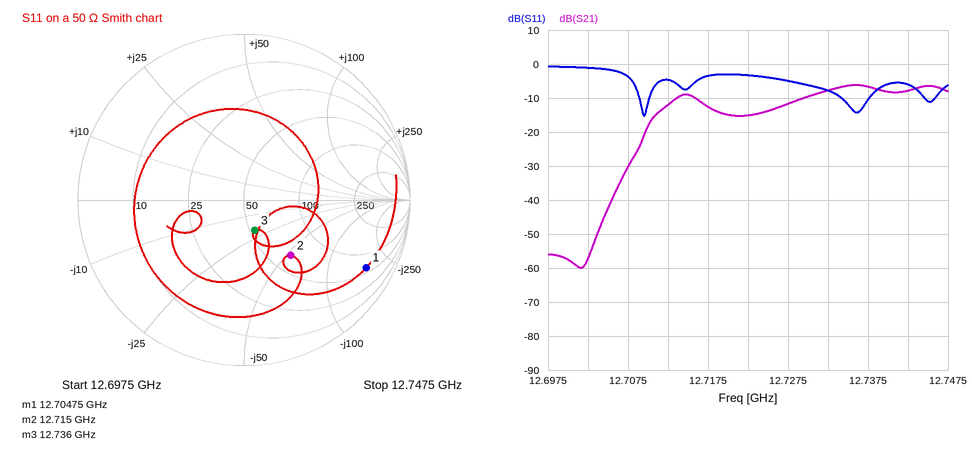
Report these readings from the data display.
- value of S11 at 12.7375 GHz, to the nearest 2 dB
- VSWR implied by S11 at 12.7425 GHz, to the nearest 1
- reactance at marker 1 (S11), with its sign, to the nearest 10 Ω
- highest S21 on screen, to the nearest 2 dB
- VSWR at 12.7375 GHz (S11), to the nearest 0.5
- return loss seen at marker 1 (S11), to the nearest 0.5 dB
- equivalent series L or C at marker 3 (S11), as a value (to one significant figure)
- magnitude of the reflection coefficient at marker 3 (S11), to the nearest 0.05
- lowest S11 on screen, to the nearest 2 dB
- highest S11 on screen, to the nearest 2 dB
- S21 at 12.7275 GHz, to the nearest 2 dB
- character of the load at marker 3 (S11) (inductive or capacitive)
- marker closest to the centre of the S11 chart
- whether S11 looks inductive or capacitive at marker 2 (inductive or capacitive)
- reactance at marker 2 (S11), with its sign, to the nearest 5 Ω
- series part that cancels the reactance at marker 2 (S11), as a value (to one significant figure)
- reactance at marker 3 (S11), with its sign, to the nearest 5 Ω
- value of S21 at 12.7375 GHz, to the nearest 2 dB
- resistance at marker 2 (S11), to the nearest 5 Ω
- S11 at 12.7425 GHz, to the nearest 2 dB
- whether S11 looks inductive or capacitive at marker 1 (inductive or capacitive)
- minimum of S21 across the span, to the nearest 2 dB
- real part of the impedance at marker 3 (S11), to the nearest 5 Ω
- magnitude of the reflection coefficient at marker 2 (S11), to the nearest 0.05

-10 dB
3
-170 Ω
-6 dB
2.0
1.5 dB
600 fF
0.20
-16 dB
0 dB
-12 dB
capacitive
marker 3
capacitive
-55 Ω
700 pH
-20 Ω
-6 dB
65 Ω
-6 dB
capacitive
-60 dB
55 Ω
0.45
